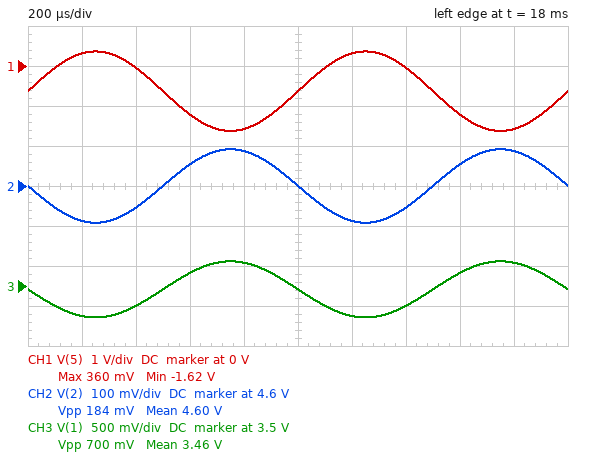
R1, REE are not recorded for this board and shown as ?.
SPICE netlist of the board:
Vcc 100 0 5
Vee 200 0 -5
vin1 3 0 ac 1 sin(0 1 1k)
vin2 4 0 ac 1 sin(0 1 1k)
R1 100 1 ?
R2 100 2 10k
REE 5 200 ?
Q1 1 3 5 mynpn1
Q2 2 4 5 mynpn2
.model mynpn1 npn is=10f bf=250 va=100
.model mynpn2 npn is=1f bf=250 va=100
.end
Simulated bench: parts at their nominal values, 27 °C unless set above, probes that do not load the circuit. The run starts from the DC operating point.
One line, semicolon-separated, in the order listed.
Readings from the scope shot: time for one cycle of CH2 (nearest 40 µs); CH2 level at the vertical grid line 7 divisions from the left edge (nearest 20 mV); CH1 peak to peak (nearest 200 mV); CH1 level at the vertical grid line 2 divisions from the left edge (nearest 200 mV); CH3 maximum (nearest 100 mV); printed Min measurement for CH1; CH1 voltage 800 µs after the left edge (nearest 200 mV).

1.00 ms; 4.54 V; 2.0 V; 0 V; 3.8 V; -1.62 V; -1.6 V
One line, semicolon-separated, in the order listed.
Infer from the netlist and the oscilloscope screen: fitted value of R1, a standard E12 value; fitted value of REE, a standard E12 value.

3.9 kΩ; 10 kΩ
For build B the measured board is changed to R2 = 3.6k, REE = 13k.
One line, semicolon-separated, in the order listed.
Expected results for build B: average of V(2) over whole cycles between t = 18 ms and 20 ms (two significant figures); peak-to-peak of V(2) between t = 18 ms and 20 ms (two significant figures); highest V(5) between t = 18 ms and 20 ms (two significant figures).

4.9 V; 51 mV; 370 mV
